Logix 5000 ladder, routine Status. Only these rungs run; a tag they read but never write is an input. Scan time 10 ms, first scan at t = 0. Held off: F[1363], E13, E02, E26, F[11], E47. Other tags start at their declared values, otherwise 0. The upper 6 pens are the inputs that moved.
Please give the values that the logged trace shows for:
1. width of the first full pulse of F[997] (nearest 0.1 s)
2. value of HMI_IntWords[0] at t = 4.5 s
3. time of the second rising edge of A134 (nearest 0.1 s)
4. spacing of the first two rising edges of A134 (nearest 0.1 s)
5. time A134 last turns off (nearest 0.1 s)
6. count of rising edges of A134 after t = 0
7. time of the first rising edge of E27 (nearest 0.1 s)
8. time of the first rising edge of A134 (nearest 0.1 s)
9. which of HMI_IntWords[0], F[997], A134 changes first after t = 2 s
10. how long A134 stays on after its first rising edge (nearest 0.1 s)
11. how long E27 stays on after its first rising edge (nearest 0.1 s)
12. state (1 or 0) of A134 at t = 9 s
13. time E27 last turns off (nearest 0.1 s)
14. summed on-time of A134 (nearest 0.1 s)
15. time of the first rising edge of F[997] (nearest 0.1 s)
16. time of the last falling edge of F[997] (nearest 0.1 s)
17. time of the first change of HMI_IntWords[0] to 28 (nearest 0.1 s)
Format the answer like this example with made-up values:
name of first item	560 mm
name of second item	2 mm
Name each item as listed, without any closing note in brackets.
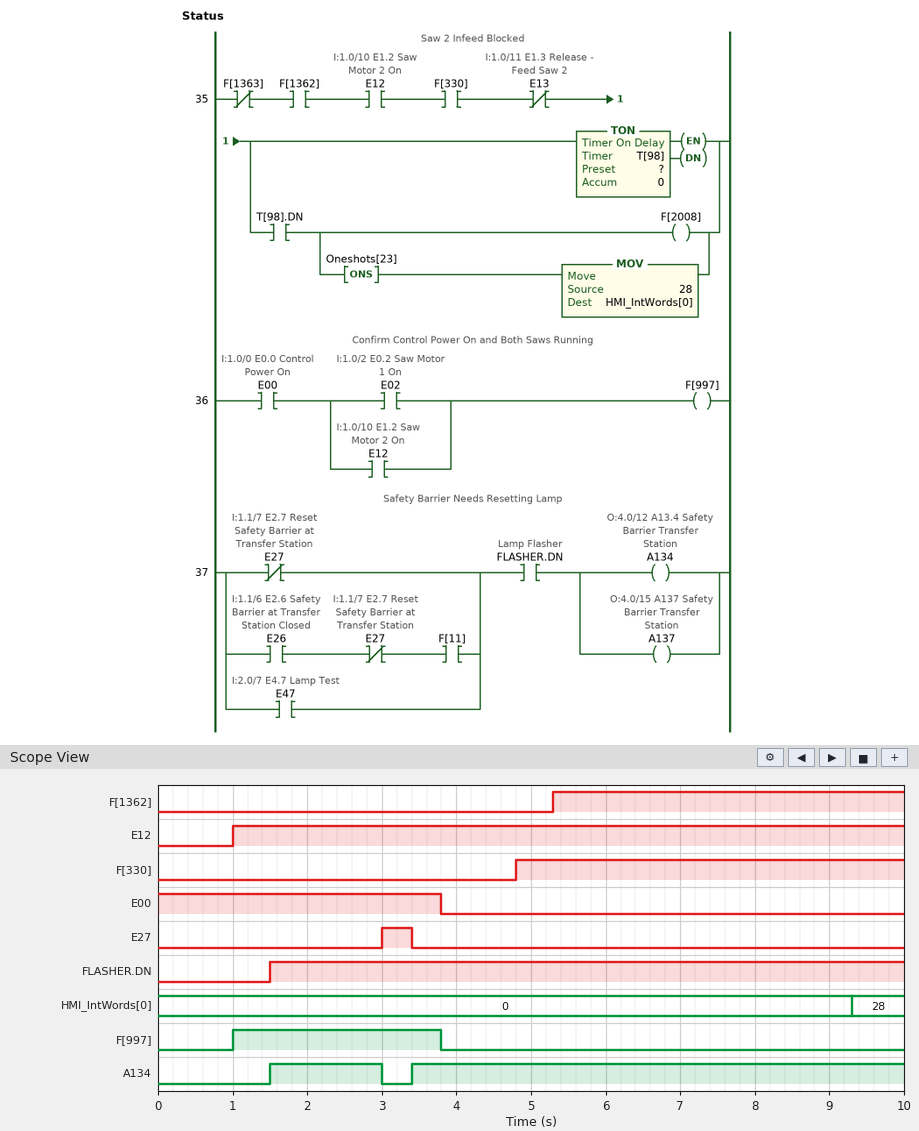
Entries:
width of the first full pulse of F[997]	2.8 s
value of HMI_IntWords[0] at t = 4.5 s	0
time of the second rising edge of A134	3.4 s
spacing of the first two rising edges of A134	1.9 s
time A134 last turns off	3.0 s
count of rising edges of A134 after t = 0	2
time of the first rising edge of E27	3.0 s
time of the first rising edge of A134	1.5 s
which of HMI_IntWords[0], F[997], A134 changes first after t = 2 s	A134
how long A134 stays on after its first rising edge	1.5 s
how long E27 stays on after its first rising edge	0.4 s
state (1 or 0) of A134 at t = 9 s	1
time E27 last turns off	3.4 s
summed on-time of A134	8.1 s
time of the first rising edge of F[997]	1.0 s
time of the last falling edge of F[997]	3.8 s
time of the first change of HMI_IntWords[0] to 28	9.3 s
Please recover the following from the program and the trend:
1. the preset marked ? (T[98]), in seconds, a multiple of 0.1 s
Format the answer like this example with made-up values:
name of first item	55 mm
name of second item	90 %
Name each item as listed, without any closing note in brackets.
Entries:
the preset marked ? (T[98]), in seconds, a multiple of 0.1 s	4.0 s
